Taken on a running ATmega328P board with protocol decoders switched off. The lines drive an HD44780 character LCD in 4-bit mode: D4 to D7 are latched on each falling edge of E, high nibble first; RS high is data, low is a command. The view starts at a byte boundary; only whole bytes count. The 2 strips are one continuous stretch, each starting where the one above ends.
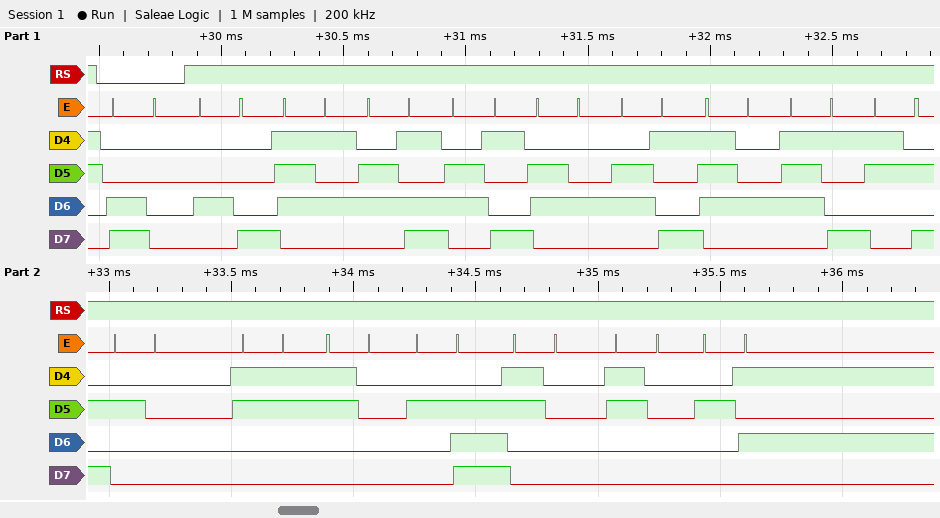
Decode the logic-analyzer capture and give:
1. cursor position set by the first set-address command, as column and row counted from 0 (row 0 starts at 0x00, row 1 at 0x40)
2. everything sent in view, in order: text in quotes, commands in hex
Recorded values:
column 0, row 1
0xC0 "Humidity: 30.00%"
